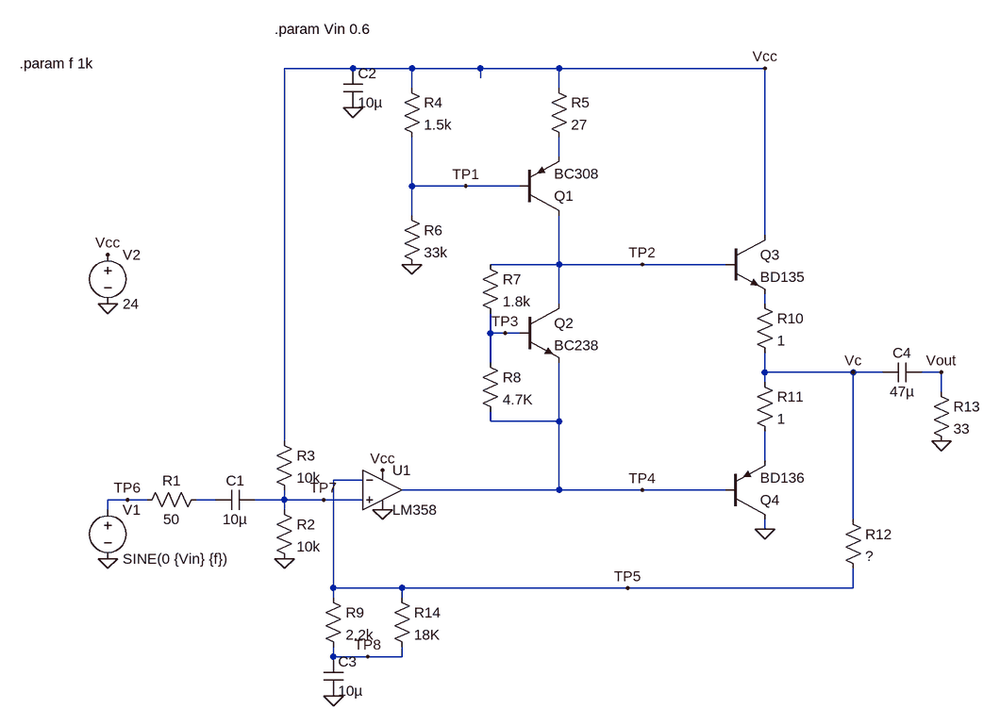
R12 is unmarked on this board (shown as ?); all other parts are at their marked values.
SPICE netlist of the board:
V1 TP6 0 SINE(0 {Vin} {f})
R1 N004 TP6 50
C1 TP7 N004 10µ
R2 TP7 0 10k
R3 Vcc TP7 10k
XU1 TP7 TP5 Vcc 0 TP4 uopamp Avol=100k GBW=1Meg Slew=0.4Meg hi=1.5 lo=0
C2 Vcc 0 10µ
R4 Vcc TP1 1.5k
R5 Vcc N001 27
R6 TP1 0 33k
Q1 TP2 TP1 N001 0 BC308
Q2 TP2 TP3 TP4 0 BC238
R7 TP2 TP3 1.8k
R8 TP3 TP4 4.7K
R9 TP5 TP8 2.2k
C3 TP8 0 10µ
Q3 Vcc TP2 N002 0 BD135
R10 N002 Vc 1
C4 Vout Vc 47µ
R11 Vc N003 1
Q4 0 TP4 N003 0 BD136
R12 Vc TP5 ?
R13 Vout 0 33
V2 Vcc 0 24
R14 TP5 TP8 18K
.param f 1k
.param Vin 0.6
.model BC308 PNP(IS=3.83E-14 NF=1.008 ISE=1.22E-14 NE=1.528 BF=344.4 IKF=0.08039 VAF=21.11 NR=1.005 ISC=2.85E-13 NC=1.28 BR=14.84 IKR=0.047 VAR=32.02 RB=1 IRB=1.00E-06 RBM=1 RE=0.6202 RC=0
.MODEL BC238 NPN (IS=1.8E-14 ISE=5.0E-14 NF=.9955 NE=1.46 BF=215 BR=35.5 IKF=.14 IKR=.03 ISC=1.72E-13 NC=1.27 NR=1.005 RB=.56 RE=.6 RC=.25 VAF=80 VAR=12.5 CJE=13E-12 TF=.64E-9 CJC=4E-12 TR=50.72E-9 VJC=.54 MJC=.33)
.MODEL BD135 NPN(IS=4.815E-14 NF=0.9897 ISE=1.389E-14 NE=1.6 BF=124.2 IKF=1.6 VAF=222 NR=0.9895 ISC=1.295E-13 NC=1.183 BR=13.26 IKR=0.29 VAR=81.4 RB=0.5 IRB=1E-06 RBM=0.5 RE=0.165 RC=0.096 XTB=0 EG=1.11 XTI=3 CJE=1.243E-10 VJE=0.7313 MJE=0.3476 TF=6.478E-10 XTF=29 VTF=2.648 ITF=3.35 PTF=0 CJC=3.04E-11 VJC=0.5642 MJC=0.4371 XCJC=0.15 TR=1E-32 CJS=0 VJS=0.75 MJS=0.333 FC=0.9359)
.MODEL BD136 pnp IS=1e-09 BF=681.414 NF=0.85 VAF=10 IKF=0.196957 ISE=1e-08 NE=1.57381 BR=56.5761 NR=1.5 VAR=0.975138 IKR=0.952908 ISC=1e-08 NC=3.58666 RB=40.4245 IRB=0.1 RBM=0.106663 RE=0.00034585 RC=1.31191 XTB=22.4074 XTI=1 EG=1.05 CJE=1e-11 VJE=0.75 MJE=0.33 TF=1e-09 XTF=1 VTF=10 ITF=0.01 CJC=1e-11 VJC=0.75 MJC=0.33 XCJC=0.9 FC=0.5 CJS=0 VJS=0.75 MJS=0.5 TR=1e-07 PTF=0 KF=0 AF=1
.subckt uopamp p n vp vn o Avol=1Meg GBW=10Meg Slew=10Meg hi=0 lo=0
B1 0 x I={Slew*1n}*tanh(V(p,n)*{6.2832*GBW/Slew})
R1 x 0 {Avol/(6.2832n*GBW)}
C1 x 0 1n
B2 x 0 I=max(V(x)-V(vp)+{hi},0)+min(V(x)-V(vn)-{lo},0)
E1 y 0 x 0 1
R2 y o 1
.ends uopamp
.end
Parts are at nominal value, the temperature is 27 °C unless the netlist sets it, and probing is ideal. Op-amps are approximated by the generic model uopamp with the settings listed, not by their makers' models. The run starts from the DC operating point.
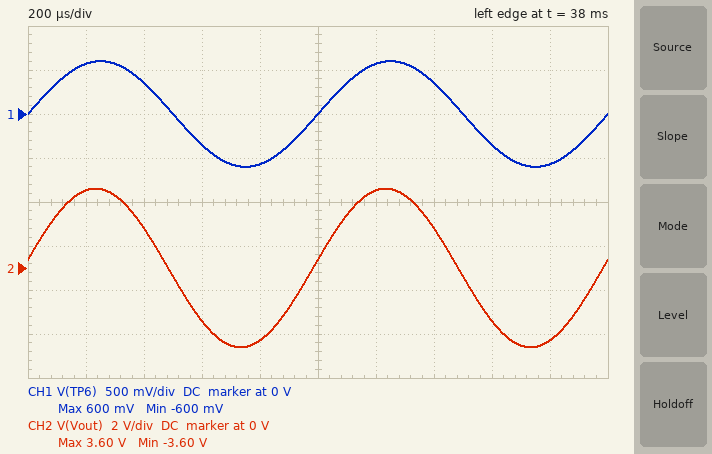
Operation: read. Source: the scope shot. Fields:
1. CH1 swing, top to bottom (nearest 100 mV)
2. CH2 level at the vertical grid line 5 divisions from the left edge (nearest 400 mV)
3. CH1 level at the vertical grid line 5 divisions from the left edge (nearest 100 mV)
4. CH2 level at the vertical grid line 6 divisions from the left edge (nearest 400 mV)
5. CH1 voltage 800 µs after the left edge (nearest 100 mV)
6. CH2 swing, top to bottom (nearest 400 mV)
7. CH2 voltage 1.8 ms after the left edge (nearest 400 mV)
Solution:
1.2 V
400 mV
0 V
3.6 V
-600 mV
7.2 V
-3.2 V
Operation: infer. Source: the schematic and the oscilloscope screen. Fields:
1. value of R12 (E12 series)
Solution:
10 kΩ
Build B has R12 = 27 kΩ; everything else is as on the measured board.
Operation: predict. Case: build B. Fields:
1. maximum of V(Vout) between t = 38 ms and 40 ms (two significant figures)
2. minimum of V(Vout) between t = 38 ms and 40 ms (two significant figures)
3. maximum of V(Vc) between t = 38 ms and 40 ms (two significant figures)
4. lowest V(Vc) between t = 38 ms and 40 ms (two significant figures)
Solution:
8.7 V
-8.7 V
21 V
3.2 V
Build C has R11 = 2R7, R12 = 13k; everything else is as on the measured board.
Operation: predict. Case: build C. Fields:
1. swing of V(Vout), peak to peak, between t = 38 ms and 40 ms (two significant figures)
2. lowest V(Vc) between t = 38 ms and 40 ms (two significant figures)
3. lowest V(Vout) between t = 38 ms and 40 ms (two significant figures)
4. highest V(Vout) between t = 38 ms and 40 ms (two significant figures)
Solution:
9.0 V
7.5 V
-4.5 V
4.5 V
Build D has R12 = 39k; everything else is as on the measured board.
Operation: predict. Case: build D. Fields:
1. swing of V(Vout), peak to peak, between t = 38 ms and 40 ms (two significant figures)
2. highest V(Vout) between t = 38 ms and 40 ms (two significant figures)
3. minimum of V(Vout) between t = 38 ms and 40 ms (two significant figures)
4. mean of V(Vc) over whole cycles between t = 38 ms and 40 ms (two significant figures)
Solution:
22 V
11 V
-11 V
12 V
